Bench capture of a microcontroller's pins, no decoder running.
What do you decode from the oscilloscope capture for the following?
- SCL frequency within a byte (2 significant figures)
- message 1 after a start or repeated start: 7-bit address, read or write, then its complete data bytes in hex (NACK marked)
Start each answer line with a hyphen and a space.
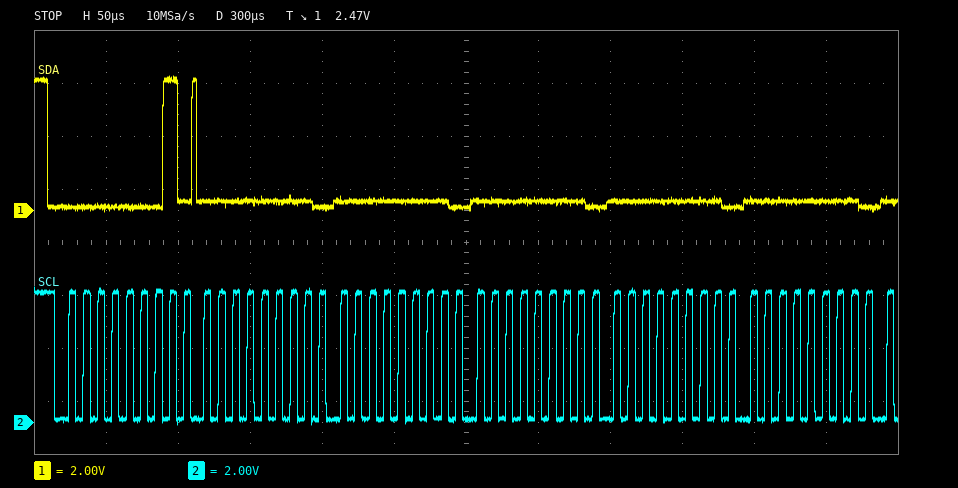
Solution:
- 100 kHz
- 0x00 read: 00 00 00 00 00
